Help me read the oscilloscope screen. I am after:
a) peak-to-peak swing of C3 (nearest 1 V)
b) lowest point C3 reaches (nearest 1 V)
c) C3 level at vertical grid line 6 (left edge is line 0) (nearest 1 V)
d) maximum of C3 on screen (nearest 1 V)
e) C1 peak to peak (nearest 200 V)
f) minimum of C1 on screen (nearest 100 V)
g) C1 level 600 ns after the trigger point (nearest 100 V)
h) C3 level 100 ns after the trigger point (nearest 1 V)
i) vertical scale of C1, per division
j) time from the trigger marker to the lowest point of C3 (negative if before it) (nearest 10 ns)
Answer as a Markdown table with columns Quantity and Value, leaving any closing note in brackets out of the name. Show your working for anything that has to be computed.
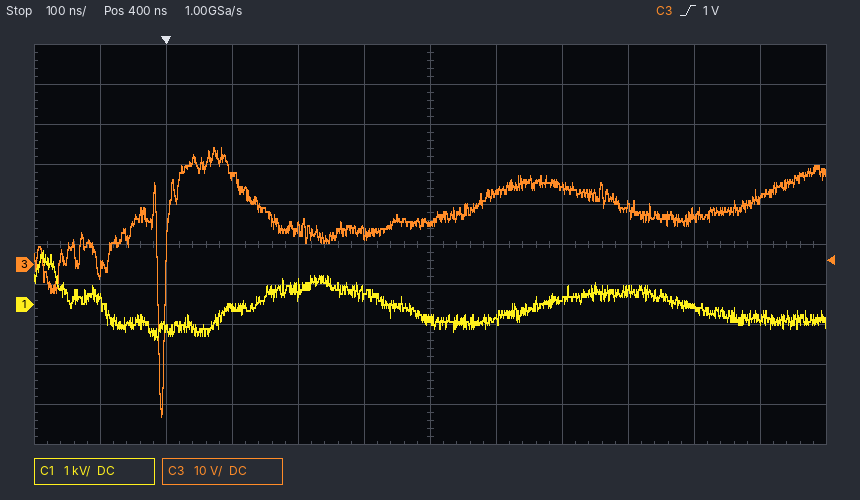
| Quantity | Value |
|---|---|
| peak-to-peak swing of C3 | 29 V − (-38 V) = 67 V |
| lowest point C3 reaches | -38 V |
| C3 level at vertical grid line 6 (left edge is line 0) | 10 V |
| maximum of C3 on screen | 29 V |
| C1 peak to peak | 2.2 kV |
| minimum of C1 on screen | -900 V |
| C1 level 600 ns after the trigger point | 100 V |
| C3 level 100 ns after the trigger point | 22 V |
| vertical scale of C1, per division | 1 kV |
| time from the trigger marker to the lowest point of C3 (negative if before it) | -10 ns |
